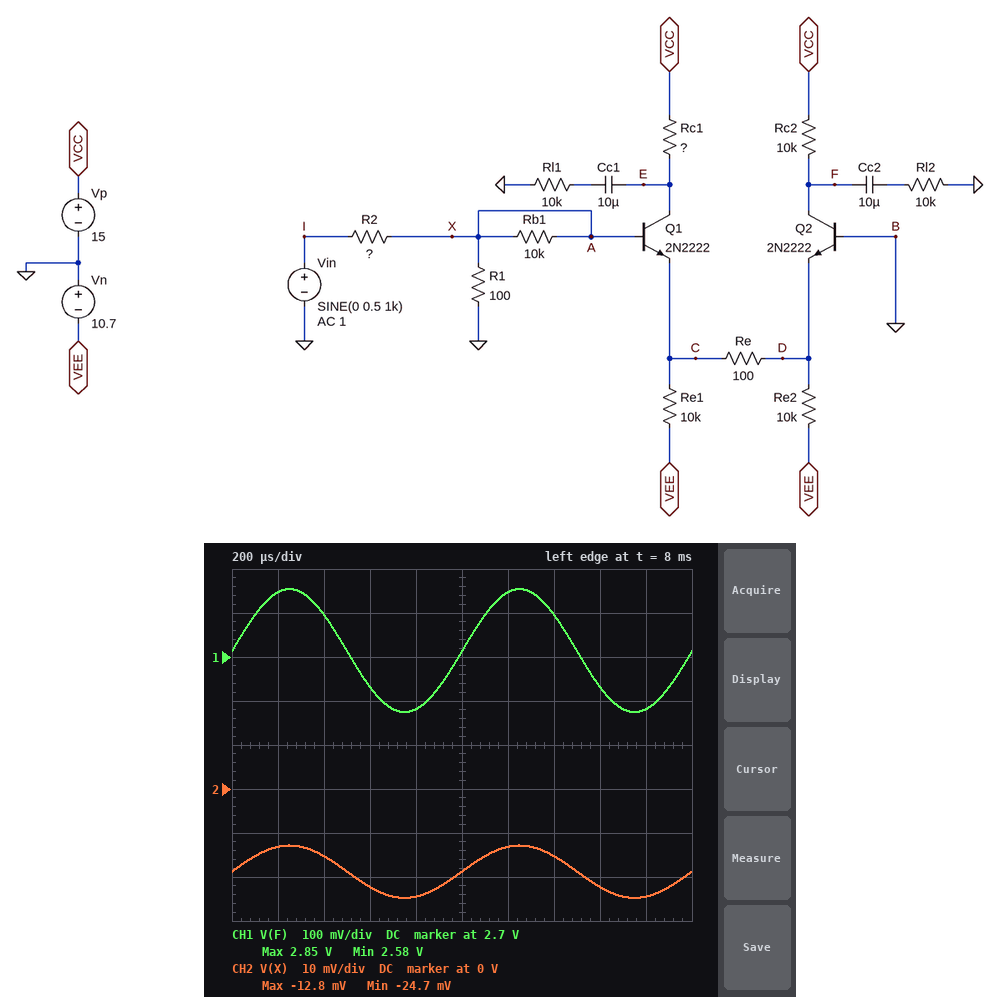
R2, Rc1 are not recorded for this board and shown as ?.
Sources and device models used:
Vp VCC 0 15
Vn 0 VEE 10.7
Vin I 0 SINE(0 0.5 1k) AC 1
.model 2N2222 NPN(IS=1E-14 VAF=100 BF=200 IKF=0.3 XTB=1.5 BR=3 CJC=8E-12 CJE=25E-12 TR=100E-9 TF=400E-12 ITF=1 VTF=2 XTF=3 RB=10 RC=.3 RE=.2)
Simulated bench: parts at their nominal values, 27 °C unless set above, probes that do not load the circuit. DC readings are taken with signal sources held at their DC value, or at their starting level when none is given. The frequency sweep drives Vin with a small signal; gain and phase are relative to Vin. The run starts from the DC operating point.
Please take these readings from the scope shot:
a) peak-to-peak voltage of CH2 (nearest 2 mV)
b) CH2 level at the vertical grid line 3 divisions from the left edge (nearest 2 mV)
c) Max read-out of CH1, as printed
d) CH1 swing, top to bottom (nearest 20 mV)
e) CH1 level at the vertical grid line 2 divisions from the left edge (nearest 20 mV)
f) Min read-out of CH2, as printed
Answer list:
12 mV
-22 mV
2.85 V
280 mV
2.80 V
-24.7 mV
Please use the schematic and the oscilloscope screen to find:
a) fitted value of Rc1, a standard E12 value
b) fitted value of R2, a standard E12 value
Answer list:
27 kΩ
5.6 kΩ
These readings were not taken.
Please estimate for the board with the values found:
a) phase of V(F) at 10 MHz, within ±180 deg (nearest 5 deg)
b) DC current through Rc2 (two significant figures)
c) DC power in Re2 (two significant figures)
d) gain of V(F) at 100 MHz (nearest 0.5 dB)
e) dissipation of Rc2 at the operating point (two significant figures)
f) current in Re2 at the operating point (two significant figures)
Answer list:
-60 deg
1.2 mA
10 mW
-35.0 dB
15 mW
1.0 mA
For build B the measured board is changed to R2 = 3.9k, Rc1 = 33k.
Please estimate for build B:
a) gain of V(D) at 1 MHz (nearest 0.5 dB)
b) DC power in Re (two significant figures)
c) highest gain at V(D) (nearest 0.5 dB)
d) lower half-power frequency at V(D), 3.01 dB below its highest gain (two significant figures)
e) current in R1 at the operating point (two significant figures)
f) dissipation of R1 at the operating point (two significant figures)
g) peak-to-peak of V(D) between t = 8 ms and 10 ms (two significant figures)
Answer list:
-53.5 dB
8.2 µW
-51.0 dB
760 kHz
230 µA
5.5 µW
1.8 mV
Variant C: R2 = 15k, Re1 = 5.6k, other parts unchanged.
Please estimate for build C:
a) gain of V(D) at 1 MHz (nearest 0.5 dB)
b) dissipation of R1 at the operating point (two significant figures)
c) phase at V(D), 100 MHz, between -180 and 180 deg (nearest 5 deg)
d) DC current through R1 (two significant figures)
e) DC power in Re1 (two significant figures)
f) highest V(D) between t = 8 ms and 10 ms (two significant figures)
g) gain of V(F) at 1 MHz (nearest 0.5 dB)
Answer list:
-61.0 dB
28 µW
-15 deg
530 µA
18 mW
-670 mV
-49.5 dB
